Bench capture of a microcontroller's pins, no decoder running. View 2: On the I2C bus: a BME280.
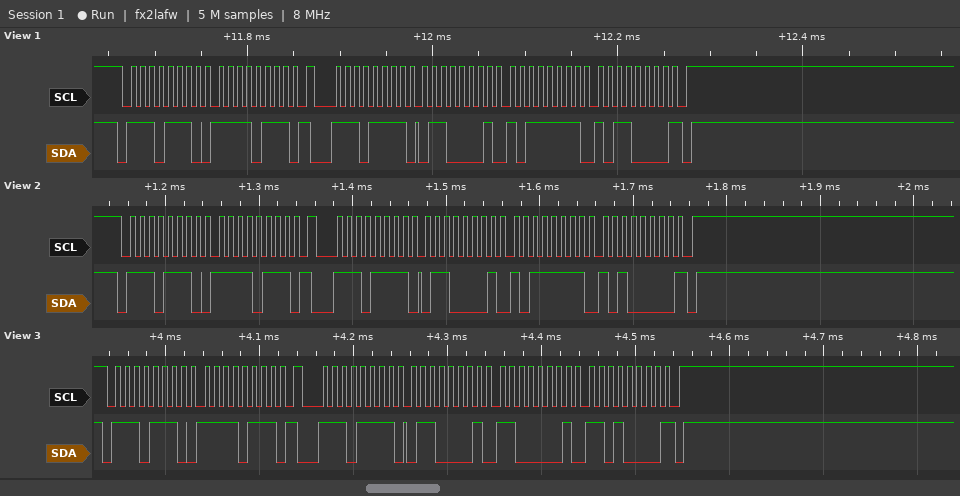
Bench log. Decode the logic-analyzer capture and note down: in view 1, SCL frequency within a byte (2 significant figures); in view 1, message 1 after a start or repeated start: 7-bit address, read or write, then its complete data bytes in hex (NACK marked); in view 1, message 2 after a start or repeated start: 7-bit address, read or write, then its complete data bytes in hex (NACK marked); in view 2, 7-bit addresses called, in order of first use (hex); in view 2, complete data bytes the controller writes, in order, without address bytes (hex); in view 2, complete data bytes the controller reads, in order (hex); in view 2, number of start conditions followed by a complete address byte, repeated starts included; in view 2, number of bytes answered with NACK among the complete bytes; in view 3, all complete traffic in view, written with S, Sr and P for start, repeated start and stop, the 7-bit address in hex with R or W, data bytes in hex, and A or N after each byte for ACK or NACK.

100 kHz
0x77 write: F7
0x77 read: 61 BF B0 NACK
0x77
F7
61 BF A0
2
1
S 77W A F7 A Sr 77R A 61 A C1 A D0 N P
